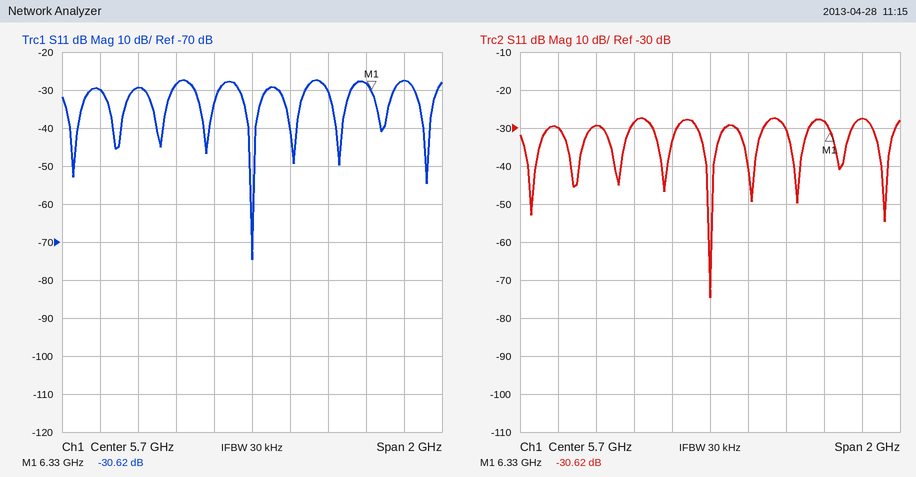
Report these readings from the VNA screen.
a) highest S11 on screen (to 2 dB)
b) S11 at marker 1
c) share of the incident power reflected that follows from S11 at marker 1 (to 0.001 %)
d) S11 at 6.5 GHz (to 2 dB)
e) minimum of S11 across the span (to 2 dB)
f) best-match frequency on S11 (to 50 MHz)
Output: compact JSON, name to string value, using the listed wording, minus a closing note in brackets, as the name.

{"highest S11 on screen": "-28 dB", "S11 at marker 1": "-30.62 dB", "share of the incident power reflected that follows from S11 at marker 1": "0.087 %", "S11 at 6.5 GHz": "-28 dB", "minimum of S11 across the span": "-74 dB", "best-match frequency on S11": "5.70 GHz"}
